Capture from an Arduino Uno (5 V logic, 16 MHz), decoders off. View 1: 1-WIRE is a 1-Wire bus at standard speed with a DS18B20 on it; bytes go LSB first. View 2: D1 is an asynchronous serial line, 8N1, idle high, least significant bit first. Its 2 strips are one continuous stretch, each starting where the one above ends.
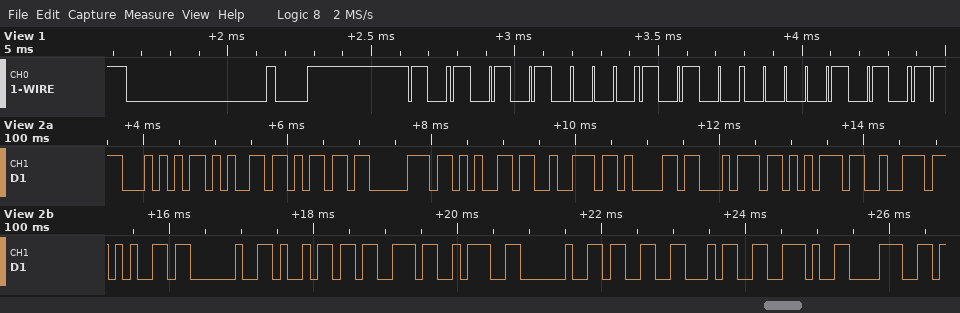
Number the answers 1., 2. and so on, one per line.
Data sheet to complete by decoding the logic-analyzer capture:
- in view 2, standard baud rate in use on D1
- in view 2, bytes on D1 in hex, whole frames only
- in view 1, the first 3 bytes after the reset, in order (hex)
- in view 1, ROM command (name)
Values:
1. 9600 baud
2. 54 65 6D 70 65 72 61 74 75 72 65 20 69 73 3A 20 33 34 2E 38
3. 55 28 50
4. Match ROM
